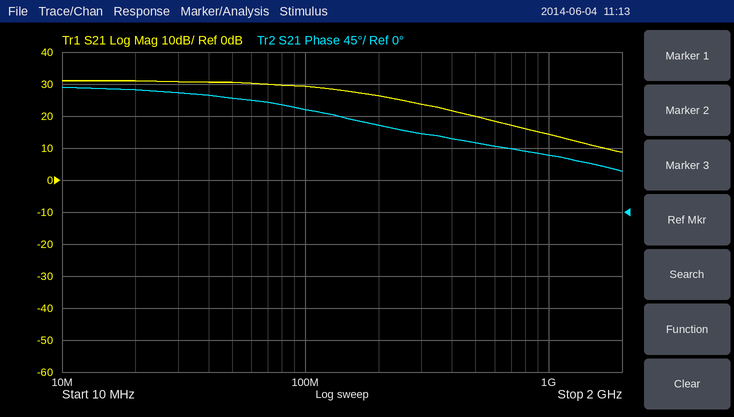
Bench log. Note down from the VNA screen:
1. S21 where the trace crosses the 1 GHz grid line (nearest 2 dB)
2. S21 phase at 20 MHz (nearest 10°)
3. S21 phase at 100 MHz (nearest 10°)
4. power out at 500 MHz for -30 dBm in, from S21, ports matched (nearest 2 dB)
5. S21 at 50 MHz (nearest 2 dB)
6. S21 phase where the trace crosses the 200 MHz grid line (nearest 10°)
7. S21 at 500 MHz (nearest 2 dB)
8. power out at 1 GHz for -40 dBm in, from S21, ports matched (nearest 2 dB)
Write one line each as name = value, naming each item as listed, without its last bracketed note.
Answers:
S21 where the trace crosses the 1 GHz grid line = 14 dB
S21 phase at 20 MHz = 170°
S21 phase at 100 MHz = 140°
power out at 500 MHz for -30 dBm in, from S21, ports matched = -10 dBm
S21 at 50 MHz = 30 dB
S21 phase where the trace crosses the 200 MHz grid line = 120°
S21 at 500 MHz = 20 dB
power out at 1 GHz for -40 dBm in, from S21, ports matched = -26 dBm
